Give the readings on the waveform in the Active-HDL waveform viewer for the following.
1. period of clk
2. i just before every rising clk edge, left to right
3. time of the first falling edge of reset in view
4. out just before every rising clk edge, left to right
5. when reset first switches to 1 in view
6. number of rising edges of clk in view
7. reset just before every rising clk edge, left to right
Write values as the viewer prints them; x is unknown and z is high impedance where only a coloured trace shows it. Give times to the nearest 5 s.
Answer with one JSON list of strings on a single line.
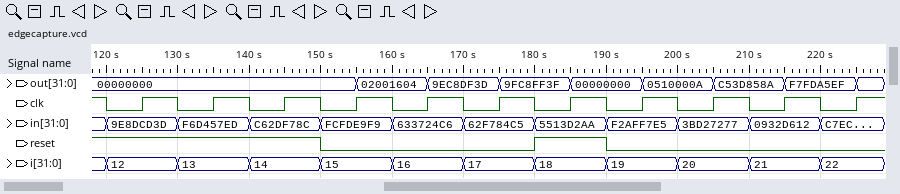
["10 s", "12, 13, 14, 15, 16, 17, 18, 19, 20, 21, 22", "150 s", "00000000, 00000000, 00000000, 00000000, 02001604, 9EC8DF3D, 9FC8FF3F, 00000000, 0510000A, C53D858A, F7FDA5EF", "180 s", "11", "1 1 1 0 0 0 1 0 0 0 0"]
